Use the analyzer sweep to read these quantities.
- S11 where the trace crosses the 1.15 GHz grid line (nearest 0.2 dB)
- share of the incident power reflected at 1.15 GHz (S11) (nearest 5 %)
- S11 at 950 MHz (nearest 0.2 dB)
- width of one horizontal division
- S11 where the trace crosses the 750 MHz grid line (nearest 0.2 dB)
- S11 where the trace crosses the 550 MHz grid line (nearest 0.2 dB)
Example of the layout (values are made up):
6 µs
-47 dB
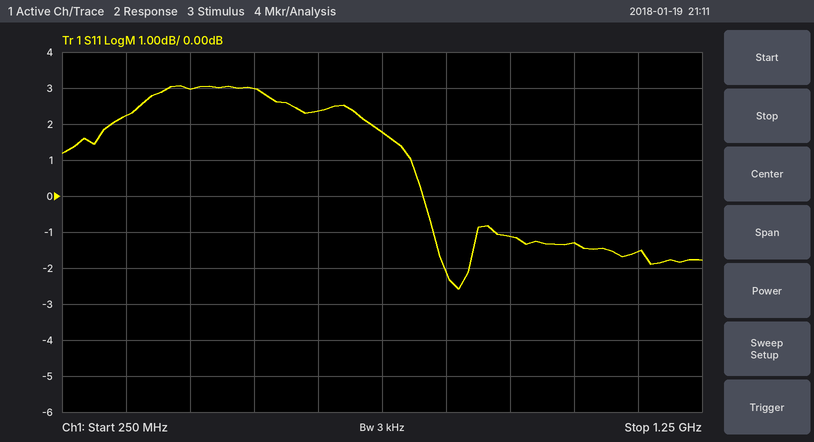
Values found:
-1.6 dB
70 %
-1.2 dB
100 MHz
1.8 dB
3.0 dB
